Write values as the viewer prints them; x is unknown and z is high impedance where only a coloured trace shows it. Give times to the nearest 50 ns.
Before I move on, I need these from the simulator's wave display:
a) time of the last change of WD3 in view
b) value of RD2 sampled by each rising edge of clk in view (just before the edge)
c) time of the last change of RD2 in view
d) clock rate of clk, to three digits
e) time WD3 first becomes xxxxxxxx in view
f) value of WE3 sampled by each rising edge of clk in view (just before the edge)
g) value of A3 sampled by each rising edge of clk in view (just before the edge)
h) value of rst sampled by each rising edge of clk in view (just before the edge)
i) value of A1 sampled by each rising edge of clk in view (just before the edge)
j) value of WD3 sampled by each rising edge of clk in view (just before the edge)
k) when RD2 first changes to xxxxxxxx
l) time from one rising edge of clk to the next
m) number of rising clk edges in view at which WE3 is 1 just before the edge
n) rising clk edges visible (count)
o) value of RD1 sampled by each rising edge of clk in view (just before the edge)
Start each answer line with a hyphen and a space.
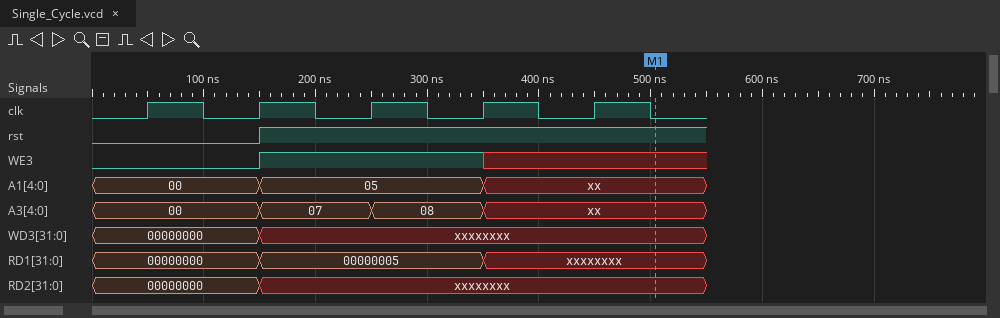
- 150 ns
- 00000000, 00000000, xxxxxxxx, xxxxxxxx, xxxxxxxx
- 150 ns
- 10.0 MHz
- 150 ns
- 0 0 1 1 x
- 00, 00, 07, 08, xx
- 0 0 1 1 1
- 00, 00, 05, 05, xx
- 00000000, 00000000, xxxxxxxx, xxxxxxxx, xxxxxxxx
- 150 ns
- 100 ns
- 2
- 5
- 00000000, 00000000, 00000005, 00000005, xxxxxxxx
